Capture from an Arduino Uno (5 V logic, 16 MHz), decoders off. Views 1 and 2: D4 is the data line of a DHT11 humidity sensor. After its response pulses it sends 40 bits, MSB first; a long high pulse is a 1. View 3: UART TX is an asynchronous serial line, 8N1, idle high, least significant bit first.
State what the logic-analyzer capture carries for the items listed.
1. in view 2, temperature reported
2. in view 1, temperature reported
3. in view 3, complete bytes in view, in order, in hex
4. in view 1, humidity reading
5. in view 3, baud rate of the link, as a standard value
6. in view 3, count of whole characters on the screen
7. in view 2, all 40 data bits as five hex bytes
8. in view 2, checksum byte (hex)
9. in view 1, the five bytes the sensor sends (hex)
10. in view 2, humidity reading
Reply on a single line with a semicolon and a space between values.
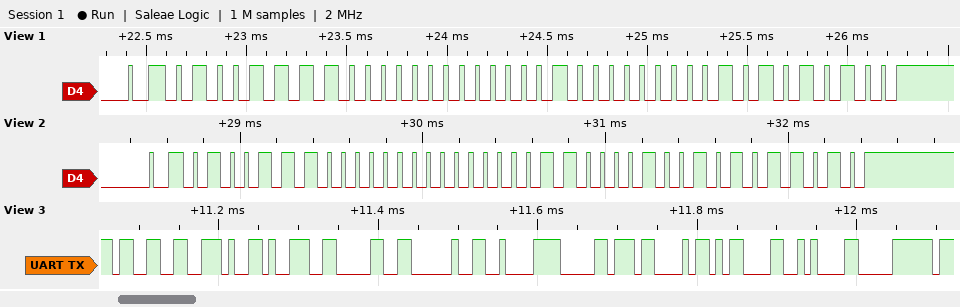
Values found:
3.9 °C; 4.1 °C; 0x33 0x2E 0x39 0x30 0x20 0xC2 0xB0 0x43 0x0D 0x0A 0xF0; 79 %; 115200 baud; 11; 4E 00 03 09 5A; 0x5A; 4F 00 04 01 54; 78 %
